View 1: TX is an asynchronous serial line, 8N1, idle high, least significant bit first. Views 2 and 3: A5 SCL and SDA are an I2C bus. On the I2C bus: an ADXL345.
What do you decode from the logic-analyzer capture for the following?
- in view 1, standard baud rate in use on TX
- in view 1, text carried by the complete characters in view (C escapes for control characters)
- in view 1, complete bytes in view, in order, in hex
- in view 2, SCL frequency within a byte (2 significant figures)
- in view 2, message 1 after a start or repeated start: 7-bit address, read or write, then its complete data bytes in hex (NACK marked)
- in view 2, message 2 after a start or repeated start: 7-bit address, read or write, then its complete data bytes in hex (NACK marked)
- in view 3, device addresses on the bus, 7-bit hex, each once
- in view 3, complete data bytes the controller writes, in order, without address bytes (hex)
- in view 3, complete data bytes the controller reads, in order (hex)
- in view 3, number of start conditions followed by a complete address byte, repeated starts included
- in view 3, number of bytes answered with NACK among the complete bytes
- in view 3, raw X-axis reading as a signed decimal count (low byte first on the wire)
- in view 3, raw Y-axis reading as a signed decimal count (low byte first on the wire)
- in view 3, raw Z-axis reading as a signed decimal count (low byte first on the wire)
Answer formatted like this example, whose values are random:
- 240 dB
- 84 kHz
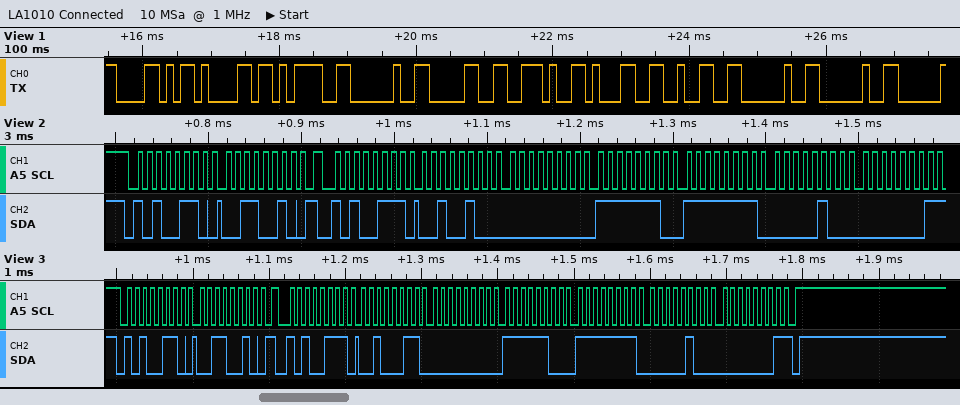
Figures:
- 9600 baud
- "Xa= 0.12  "
- 0x58 0x61 0x3D 0x20 0x30 0x2E 0x31 0x32 0x20 0x20
- 100 kHz
- 0x53 write: 32
- 0x53 read: 24 00 FE FF 04 01 NACK
- 0x53
- 32
- 23 00 FC FF 04 01
- 2
- 1
- 35
- -4
- 260
